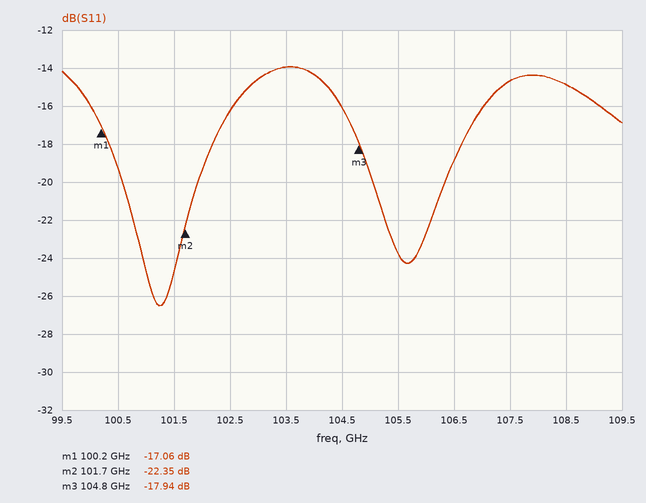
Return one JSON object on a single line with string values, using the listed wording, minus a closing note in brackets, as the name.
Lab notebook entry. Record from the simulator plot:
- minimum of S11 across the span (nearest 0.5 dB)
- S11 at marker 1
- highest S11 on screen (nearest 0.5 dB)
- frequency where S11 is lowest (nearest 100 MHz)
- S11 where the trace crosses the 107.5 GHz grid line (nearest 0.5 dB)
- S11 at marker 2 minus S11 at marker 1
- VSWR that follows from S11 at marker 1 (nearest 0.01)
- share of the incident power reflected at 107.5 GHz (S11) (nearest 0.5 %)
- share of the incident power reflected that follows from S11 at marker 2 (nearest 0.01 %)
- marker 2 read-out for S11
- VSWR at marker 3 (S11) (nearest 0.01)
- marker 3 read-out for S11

{"minimum of S11 across the span": "-26.5 dB", "S11 at marker 1": "-17.06 dB", "highest S11 on screen": "-14.0 dB", "frequency where S11 is lowest": "101.2 GHz", "S11 where the trace crosses the 107.5 GHz grid line": "-14.5 dB", "S11 at marker 2 minus S11 at marker 1": "-5.29 dB", "VSWR that follows from S11 at marker 1": "1.33", "share of the incident power reflected at 107.5 GHz (S11)": "3.5 %", "share of the incident power reflected that follows from S11 at marker 2": "0.58 %", "marker 2 read-out for S11": "-22.35 dB", "VSWR at marker 3 (S11)": "1.29", "marker 3 read-out for S11": "-17.94 dB"}
